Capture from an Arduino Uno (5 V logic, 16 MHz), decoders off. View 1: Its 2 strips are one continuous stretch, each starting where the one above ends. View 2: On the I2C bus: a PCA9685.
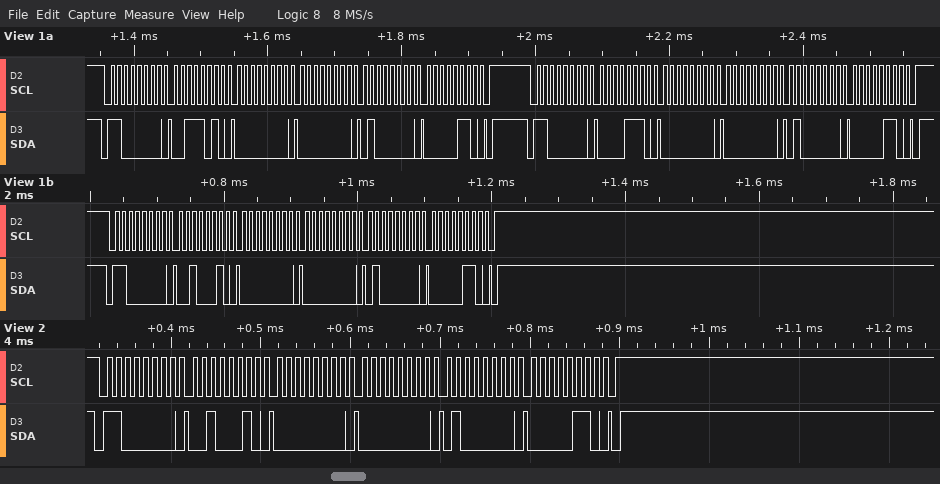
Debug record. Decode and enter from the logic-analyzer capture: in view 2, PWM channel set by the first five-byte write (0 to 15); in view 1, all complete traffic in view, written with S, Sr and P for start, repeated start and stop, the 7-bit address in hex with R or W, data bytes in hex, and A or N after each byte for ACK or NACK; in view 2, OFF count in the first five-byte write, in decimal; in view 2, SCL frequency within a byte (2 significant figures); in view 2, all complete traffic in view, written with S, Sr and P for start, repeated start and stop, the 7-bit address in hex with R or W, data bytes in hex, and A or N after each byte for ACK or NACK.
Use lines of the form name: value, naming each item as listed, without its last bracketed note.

in view 2, PWM channel set by the first five-byte write: 7
in view 1, all complete traffic in view, written with S, Sr and P for start, repeated start and stop, the 7-bit address in hex with R or W, data bytes in hex, and A or N after each byte for ACK or NACK: S 60W A 3A A 00 A 00 A 40 A 06 A P S 60W A 0E A 00 A 00 A 40 A 06 A P S 60W A 22 A 00 A 00 A 40 A 06 A P
in view 2, OFF count in the first five-byte write, in decimal: 1600
in view 2, SCL frequency within a byte: 100 kHz
in view 2, all complete traffic in view, written with S, Sr and P for start, repeated start and stop, the 7-bit address in hex with R or W, data bytes in hex, and A or N after each byte for ACK or NACK: S 60W A 22 A 00 A 00 A 40 A 06 A P
